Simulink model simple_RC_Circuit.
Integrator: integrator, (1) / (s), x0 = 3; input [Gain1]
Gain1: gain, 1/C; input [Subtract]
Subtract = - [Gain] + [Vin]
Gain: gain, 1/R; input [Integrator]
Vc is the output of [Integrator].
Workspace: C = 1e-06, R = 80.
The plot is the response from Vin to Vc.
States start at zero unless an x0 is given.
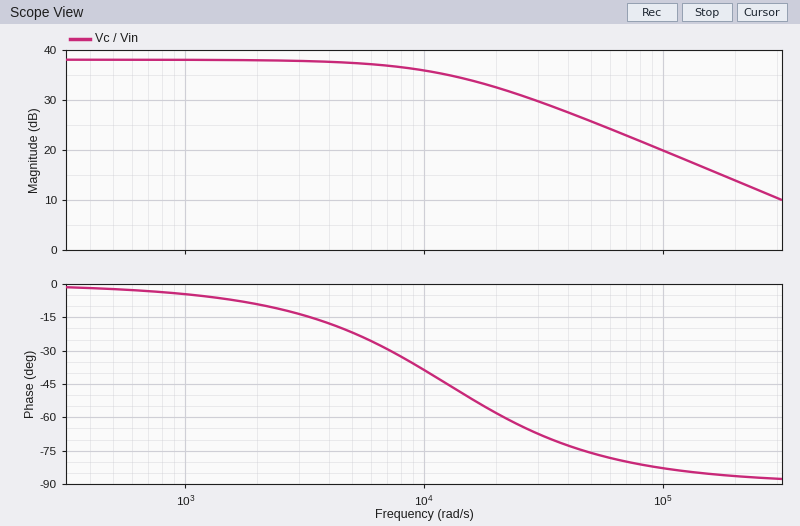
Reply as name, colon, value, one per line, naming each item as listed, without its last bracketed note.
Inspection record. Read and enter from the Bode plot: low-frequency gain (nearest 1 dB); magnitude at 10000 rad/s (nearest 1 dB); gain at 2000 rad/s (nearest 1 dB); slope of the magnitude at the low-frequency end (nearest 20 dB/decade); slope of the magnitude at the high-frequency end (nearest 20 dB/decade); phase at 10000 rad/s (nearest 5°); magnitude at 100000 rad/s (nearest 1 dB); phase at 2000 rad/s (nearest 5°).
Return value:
low-frequency gain: 38 dB
magnitude at 10000 rad/s: 36 dB
gain at 2000 rad/s: 38 dB
slope of the magnitude at the low-frequency end: 0 dB/decade
slope of the magnitude at the high-frequency end: -20 dB/decade
phase at 10000 rad/s: -40°
magnitude at 100000 rad/s: 20 dB
phase at 2000 rad/s: -10°
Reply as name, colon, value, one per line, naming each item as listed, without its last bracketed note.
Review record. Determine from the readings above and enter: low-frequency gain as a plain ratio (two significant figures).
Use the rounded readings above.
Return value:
low-frequency gain as a plain ratio: 79
